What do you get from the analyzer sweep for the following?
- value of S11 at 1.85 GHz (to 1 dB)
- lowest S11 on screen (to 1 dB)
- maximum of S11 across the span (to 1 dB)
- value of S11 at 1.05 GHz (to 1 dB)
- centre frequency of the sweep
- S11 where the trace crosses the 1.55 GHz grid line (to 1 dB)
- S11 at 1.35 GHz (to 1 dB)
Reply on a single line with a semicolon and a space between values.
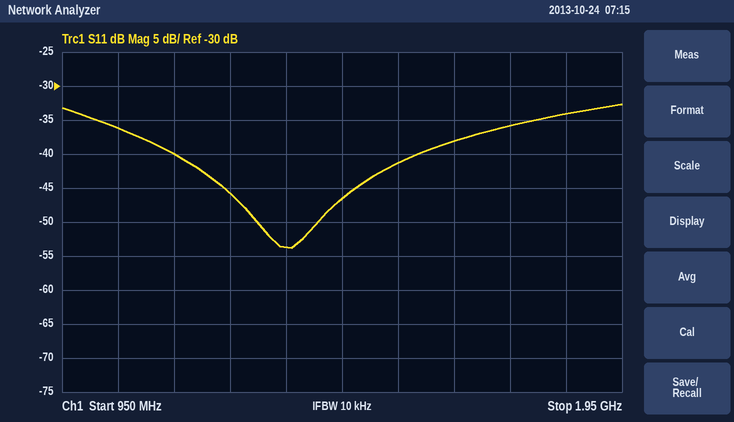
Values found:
-34 dB; -54 dB; -33 dB; -36 dB; 1.45 GHz; -41 dB; -54 dB
